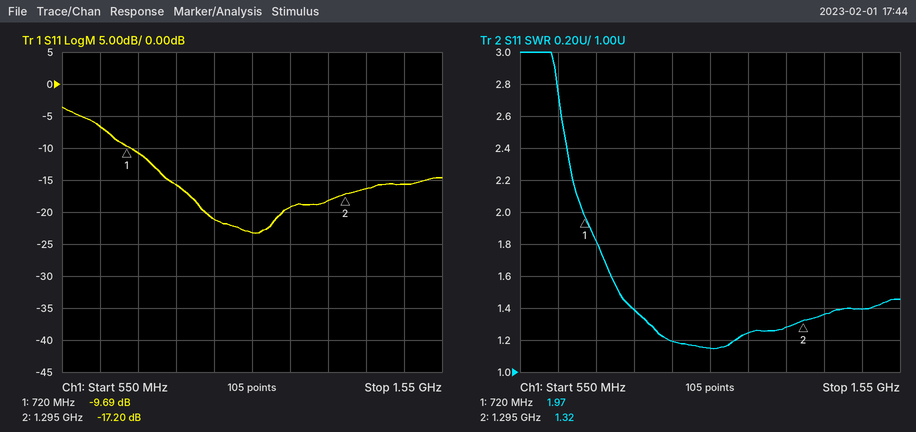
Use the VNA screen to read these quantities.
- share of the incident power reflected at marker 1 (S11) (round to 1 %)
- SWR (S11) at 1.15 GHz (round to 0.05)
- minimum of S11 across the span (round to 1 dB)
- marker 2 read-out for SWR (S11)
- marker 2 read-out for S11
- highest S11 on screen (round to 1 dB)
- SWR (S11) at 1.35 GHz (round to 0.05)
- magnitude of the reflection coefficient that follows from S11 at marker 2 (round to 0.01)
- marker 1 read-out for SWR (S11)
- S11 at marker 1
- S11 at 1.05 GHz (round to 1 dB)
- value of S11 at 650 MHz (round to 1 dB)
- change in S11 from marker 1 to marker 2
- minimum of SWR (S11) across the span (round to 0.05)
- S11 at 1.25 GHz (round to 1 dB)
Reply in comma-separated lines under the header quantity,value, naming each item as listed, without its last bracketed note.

quantity,value
share of the incident power reflected at marker 1 (S11),11 %
SWR (S11) at 1.15 GHz,1.25
minimum of S11 across the span,-23 dB
marker 2 read-out for SWR,1.32
marker 2 read-out for S11,-17.20 dB
highest S11 on screen,-4 dB
SWR (S11) at 1.35 GHz,1.35
magnitude of the reflection coefficient that follows from S11 at marker 2,0.14
marker 1 read-out for SWR,1.97
S11 at marker 1,-9.69 dB
S11 at 1.05 GHz,-23 dB
value of S11 at 650 MHz,-7 dB
change in S11 from marker 1 to marker 2,-7.51 dB
minimum of SWR (S11) across the span,1.15
S11 at 1.25 GHz,-18 dB
